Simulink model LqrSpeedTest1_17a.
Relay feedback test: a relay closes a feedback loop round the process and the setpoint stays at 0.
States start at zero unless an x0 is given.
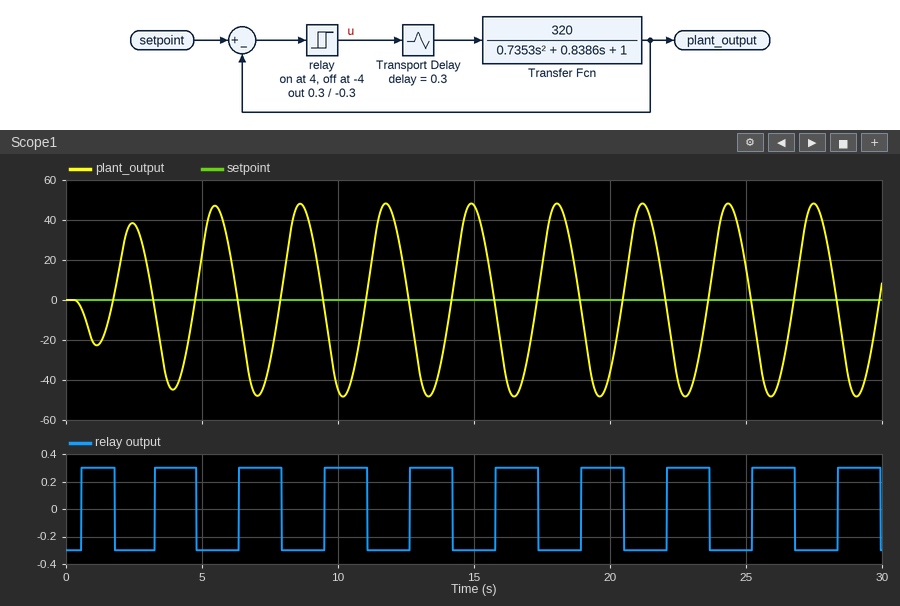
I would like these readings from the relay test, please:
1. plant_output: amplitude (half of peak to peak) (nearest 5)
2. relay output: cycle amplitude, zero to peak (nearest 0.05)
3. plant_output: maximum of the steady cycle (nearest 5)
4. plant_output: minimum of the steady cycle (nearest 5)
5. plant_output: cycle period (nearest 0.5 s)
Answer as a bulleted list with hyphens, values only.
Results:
- 50
- 0.30
- 50
- -50
- 3.0 s
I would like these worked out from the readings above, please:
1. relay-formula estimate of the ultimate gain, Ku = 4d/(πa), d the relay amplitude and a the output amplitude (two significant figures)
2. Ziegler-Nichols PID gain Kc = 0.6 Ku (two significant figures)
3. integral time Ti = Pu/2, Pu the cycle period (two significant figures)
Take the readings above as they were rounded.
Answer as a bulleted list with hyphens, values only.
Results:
- 0.0076
- 0.0046
- 1.5 s
